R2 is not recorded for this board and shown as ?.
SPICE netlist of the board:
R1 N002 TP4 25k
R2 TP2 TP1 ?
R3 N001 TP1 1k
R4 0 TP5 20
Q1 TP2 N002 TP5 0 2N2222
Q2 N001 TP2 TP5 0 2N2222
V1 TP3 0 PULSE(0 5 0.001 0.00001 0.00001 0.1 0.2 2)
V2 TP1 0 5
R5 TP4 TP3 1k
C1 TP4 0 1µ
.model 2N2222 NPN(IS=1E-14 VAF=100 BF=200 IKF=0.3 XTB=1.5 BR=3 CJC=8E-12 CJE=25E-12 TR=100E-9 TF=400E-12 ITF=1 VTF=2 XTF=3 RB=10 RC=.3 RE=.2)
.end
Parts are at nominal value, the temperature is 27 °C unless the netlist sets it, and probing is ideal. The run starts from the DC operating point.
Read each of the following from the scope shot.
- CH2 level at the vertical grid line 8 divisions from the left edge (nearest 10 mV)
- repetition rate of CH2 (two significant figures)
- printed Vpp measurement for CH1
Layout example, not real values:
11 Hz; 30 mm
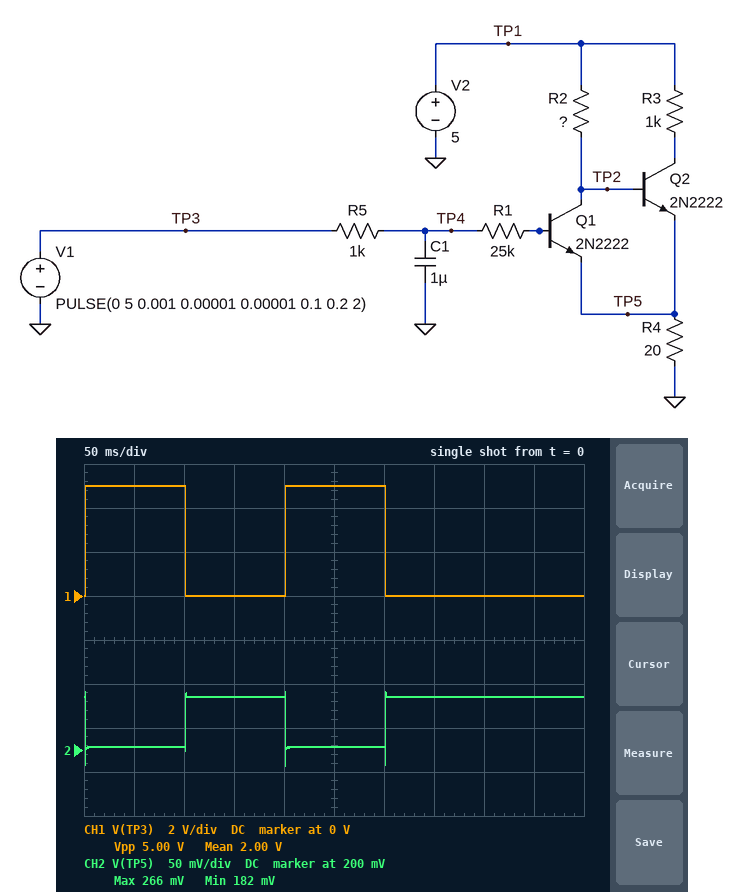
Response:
260 mV; 5.0 Hz; 5.00 V
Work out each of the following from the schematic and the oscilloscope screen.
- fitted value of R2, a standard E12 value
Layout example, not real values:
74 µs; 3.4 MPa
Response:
470 Ω
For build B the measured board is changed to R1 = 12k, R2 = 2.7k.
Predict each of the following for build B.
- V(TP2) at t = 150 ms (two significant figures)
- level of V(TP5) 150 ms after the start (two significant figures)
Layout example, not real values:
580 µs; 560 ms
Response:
860 mV; 130 mV
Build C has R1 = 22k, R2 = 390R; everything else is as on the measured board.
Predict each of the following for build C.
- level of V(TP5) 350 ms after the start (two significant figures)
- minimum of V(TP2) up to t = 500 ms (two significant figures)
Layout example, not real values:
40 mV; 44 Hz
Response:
290 mV; 340 mV
